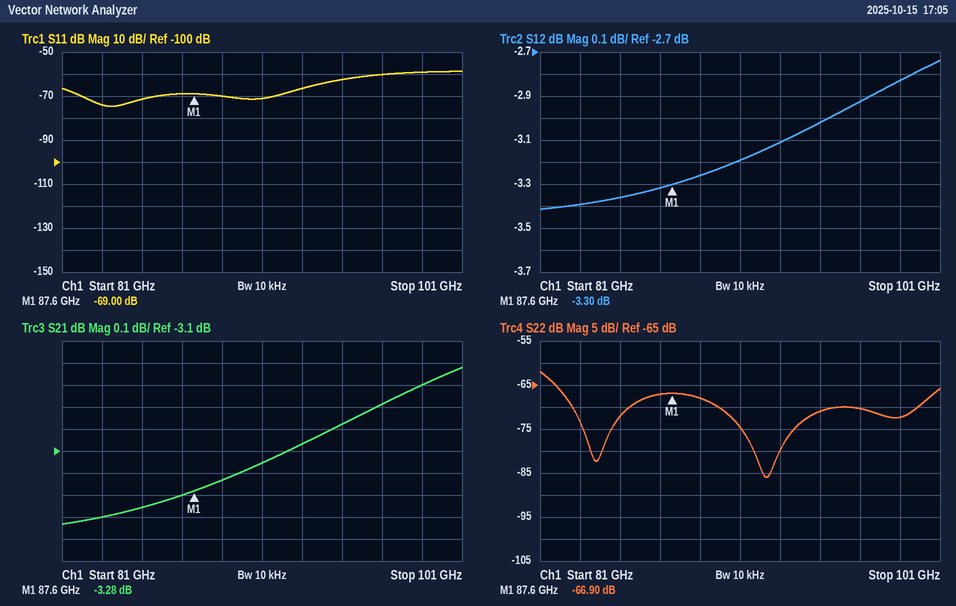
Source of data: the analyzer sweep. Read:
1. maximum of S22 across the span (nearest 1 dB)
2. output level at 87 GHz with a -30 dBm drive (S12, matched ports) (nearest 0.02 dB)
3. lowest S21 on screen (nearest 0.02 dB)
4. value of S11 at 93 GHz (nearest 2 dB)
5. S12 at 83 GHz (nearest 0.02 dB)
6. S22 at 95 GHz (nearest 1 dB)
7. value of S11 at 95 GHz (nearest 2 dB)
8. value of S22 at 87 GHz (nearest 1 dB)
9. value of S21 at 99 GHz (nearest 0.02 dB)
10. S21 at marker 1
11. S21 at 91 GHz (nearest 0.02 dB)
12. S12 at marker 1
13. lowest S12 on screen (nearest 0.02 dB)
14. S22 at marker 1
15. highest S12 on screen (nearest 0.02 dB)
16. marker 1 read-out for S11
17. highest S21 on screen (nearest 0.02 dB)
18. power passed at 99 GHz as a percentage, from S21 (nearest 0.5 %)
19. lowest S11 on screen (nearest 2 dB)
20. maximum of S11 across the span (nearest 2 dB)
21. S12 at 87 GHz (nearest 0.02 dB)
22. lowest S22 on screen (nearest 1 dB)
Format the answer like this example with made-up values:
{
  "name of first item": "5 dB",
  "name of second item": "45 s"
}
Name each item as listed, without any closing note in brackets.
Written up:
{
  "maximum of S22 across the span": "-62 dB",
  "output level at 87 GHz with a -30 dBm drive (S12, matched ports)": "-33.32 dBm",
  "lowest S21 on screen": "-3.44 dB",
  "value of S11 at 93 GHz": "-66 dB",
  "S12 at 83 GHz": "-3.40 dB",
  "S22 at 95 GHz": "-71 dB",
  "value of S11 at 95 GHz": "-62 dB",
  "value of S22 at 87 GHz": "-67 dB",
  "value of S21 at 99 GHz": "-2.80 dB",
  "S21 at marker 1": "-3.28 dB",
  "S21 at 91 GHz": "-3.16 dB",
  "S12 at marker 1": "-3.30 dB",
  "lowest S12 on screen": "-3.42 dB",
  "S22 at marker 1": "-66.90 dB",
  "highest S12 on screen": "-2.74 dB",
  "marker 1 read-out for S11": "-69.00 dB",
  "highest S21 on screen": "-2.72 dB",
  "power passed at 99 GHz as a percentage, from S21": "52.5 %",
  "lowest S11 on screen": "-74 dB",
  "maximum of S11 across the span": "-58 dB",
  "S12 at 87 GHz": "-3.32 dB",
  "lowest S22 on screen": "-86 dB"
}
